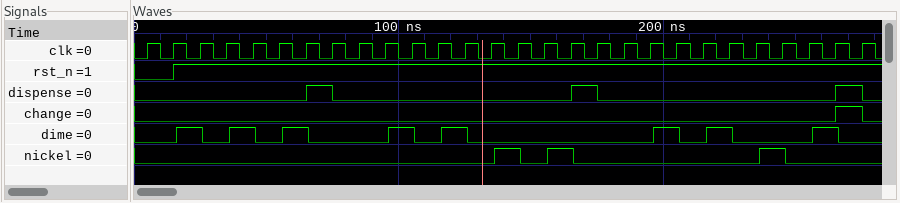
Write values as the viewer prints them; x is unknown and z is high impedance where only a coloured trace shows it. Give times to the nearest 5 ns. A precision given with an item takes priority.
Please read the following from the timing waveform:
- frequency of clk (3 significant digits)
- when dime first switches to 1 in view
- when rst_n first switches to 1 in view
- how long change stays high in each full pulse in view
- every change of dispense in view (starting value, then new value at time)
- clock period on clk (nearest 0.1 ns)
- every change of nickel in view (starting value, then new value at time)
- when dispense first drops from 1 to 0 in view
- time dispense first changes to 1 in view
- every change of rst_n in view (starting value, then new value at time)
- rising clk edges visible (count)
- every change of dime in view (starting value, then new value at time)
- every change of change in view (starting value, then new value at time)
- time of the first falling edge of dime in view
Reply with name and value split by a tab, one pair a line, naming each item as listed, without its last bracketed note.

frequency of clk	100 MHz
when dime first switches to 1 in view	15 ns
when rst_n first switches to 1 in view	15 ns
how long change stays high in each full pulse in view	10 ns
every change of dispense in view	0, 1 at 65 ns, 0 at 75 ns, 1 at 165 ns, 0 at 175 ns, 1 at 265 ns, 0 at 275 ns
clock period on clk	10 ns
every change of nickel in view	0, 1 at 135 ns, 0 at 145 ns, 1 at 155 ns, 0 at 165 ns, 1 at 235 ns, 0 at 245 ns
when dispense first drops from 1 to 0 in view	75 ns
time dispense first changes to 1 in view	65 ns
every change of rst_n in view	0, 1 at 15 ns
rising clk edges visible	28
every change of dime in view	0, 1 at 15 ns, 0 at 25 ns, 1 at 35 ns, 0 at 45 ns, 1 at 55 ns, 0 at 65 ns, 1 at 95 ns, 0 at 105 ns, 1 at 115 ns, 0 at 125 ns, 1 at 195 ns, 0 at 205 ns, 1 at 215 ns, 0 at 225 ns, 1 at 255 ns, 0 at 265 ns
every change of change in view	0, 1 at 265 ns, 0 at 275 ns
time of the first falling edge of dime in view	25 ns
